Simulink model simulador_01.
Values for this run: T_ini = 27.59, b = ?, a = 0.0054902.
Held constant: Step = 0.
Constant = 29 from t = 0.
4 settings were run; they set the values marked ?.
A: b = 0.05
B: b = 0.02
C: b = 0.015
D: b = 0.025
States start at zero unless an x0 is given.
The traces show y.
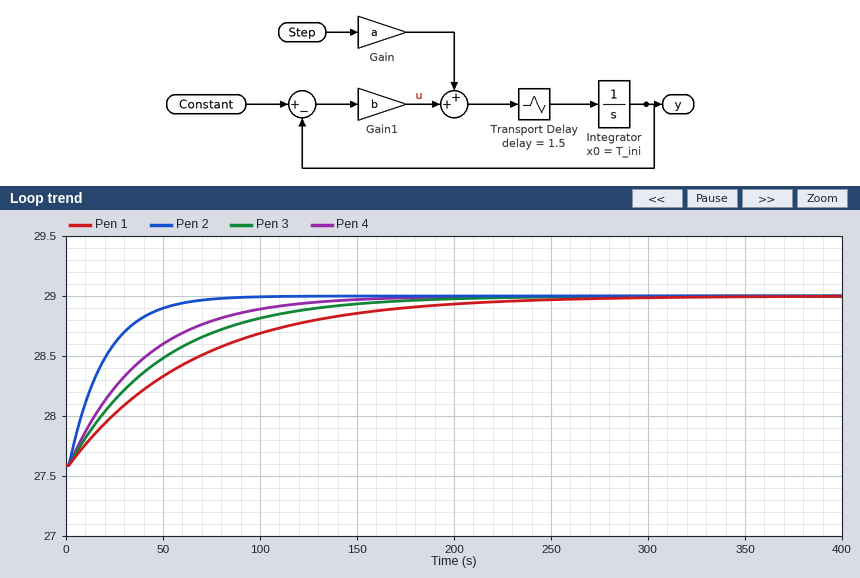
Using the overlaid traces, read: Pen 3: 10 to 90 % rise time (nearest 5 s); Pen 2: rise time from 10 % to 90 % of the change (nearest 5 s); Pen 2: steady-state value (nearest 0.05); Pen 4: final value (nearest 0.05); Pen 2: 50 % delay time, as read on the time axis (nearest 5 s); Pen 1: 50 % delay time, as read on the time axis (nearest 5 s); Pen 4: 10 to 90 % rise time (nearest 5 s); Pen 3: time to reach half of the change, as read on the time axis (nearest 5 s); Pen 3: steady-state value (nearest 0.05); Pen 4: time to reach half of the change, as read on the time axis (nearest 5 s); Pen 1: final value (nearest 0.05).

105 s
40 s
29.00
29.00
15 s
45 s
85 s
35 s
29.00
30 s
29.00
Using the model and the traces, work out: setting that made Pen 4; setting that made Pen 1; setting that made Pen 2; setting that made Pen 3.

D
C
A
B
